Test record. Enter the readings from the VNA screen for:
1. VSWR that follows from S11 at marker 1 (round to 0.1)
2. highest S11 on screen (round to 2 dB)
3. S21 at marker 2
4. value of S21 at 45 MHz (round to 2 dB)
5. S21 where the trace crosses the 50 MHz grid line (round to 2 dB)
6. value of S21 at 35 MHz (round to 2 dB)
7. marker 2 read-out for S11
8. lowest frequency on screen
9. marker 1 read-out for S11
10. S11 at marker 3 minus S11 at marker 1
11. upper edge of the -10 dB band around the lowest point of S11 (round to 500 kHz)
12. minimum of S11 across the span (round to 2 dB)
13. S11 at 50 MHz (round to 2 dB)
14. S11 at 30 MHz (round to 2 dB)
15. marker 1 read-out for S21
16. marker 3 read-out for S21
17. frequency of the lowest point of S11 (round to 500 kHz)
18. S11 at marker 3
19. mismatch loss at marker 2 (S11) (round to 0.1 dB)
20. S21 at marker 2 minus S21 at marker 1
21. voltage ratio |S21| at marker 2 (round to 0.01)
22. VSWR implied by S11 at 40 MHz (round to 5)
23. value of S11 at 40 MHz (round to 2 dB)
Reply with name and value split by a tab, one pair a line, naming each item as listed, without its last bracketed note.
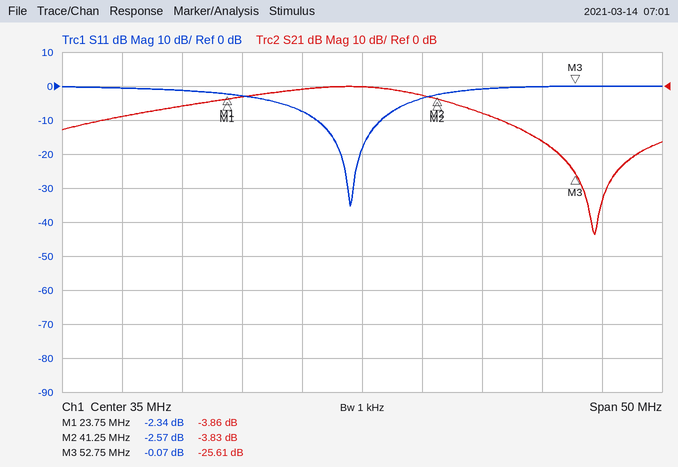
VSWR that follows from S11 at marker 1	7.5
highest S11 on screen	0 dB
S21 at marker 2	-3.83 dB
value of S21 at 45 MHz	-8 dB
S21 where the trace crosses the 50 MHz grid line	-16 dB
value of S21 at 35 MHz	0 dB
marker 2 read-out for S11	-2.57 dB
lowest frequency on screen	10 MHz
marker 1 read-out for S11	-2.34 dB
S11 at marker 3 minus S11 at marker 1	2.27 dB
upper edge of the -10 dB band around the lowest point of S11	36.5 MHz
minimum of S11 across the span	-36 dB
S11 at 50 MHz	0 dB
S11 at 30 MHz	-8 dB
marker 1 read-out for S21	-3.86 dB
marker 3 read-out for S21	-25.61 dB
frequency of the lowest point of S11	34.0 MHz
S11 at marker 3	-0.07 dB
mismatch loss at marker 2 (S11)	3.5 dB
S21 at marker 2 minus S21 at marker 1	0.03 dB
voltage ratio |S21| at marker 2	0.64
VSWR implied by S11 at 40 MHz	5
value of S11 at 40 MHz	-4 dB
